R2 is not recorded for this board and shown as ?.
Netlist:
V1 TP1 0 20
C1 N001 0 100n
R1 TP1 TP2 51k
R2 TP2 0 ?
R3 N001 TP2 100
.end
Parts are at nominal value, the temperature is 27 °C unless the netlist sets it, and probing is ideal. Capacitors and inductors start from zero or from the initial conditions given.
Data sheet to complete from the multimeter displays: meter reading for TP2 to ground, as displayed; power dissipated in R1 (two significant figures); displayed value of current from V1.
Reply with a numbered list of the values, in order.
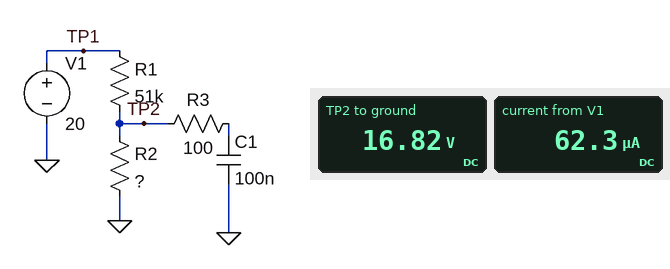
1. 16.82 V
2. 200 µW
3. 62.3 µA
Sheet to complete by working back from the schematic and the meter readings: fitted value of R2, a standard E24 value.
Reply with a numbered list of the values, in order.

1. 270 kΩ
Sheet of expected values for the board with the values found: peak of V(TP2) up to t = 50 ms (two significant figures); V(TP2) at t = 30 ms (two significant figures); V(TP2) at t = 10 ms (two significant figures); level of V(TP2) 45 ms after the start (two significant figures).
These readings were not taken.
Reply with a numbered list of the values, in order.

1. 17 V
2. 17 V
3. 15 V
4. 17 V
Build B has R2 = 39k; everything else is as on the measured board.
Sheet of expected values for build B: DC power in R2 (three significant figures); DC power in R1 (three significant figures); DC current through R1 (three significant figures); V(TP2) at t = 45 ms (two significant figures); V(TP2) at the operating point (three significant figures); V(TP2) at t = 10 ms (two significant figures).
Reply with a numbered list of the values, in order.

1. 1.93 mW
2. 2.52 mW
3. 222 µA
4. 8.7 V
5. 8.67 V
6. 8.6 V
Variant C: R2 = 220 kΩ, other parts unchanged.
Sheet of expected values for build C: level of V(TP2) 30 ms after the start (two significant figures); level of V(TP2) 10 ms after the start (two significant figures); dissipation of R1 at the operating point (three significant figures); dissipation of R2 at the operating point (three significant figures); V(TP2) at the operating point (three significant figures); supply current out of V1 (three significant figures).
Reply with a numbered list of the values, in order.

1. 16 V
2. 15 V
3. 278 µW
4. 1.20 mW
5. 16.2 V
6. 73.8 µA
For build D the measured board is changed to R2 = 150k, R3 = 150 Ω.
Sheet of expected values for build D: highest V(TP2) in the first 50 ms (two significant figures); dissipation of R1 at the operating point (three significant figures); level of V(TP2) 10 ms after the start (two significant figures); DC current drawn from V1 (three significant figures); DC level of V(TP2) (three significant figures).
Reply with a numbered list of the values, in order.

1. 15 V
2. 505 µW
3. 14 V
4. 99.5 µA
5. 14.9 V
